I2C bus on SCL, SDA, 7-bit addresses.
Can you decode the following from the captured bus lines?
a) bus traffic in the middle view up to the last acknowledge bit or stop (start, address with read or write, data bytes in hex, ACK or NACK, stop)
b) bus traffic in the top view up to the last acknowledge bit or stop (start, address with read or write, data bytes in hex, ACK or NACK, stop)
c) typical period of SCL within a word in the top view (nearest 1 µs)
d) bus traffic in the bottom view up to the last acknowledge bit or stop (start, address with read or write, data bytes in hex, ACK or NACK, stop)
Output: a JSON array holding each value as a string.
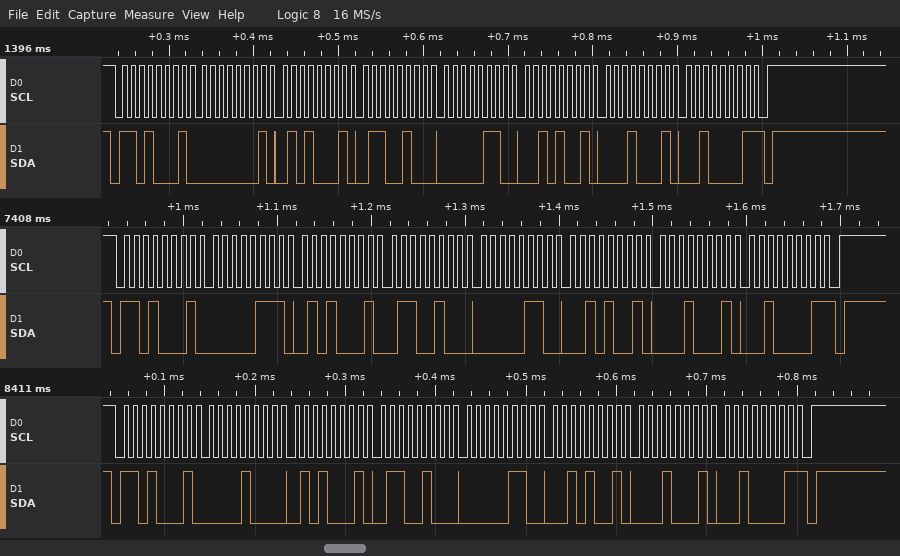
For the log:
["start, address 68 read ACK, 07 ACK, 51 ACK, 64 ACK, 06 ACK, 29 ACK, 11 ACK, 21 NACK, stop", "start, address 68 read ACK, 01 ACK, 51 ACK, 64 ACK, 06 ACK, 29 ACK, 11 ACK, 21 NACK, stop", "10 µs", "start, address 68 read ACK, 08 ACK, 51 ACK, 64 ACK, 06 ACK, 29 ACK, 11 ACK, 21 NACK, stop"]
